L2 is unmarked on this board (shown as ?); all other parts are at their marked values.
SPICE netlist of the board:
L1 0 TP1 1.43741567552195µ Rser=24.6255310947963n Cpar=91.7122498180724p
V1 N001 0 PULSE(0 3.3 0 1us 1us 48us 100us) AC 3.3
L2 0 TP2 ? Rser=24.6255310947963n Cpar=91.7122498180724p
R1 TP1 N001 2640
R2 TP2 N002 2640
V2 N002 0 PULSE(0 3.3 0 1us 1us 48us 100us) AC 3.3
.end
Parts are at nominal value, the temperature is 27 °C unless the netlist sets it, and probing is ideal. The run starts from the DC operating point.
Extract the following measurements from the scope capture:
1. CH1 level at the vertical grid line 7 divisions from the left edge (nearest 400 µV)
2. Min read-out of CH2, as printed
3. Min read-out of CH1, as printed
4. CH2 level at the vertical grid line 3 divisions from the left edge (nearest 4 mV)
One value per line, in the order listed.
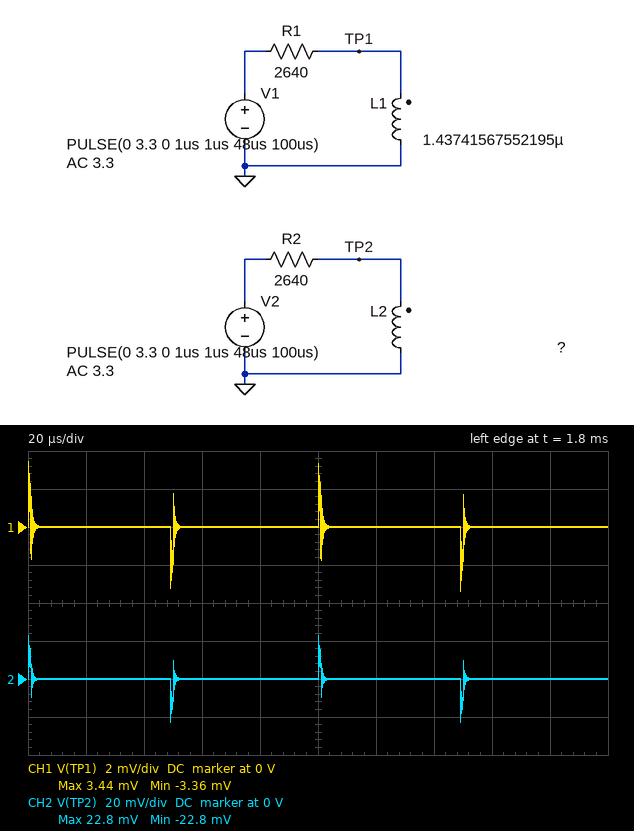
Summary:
0 V
-22.8 mV
-3.36 mV
0 V
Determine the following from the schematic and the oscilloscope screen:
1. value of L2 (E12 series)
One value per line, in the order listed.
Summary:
10 µH
